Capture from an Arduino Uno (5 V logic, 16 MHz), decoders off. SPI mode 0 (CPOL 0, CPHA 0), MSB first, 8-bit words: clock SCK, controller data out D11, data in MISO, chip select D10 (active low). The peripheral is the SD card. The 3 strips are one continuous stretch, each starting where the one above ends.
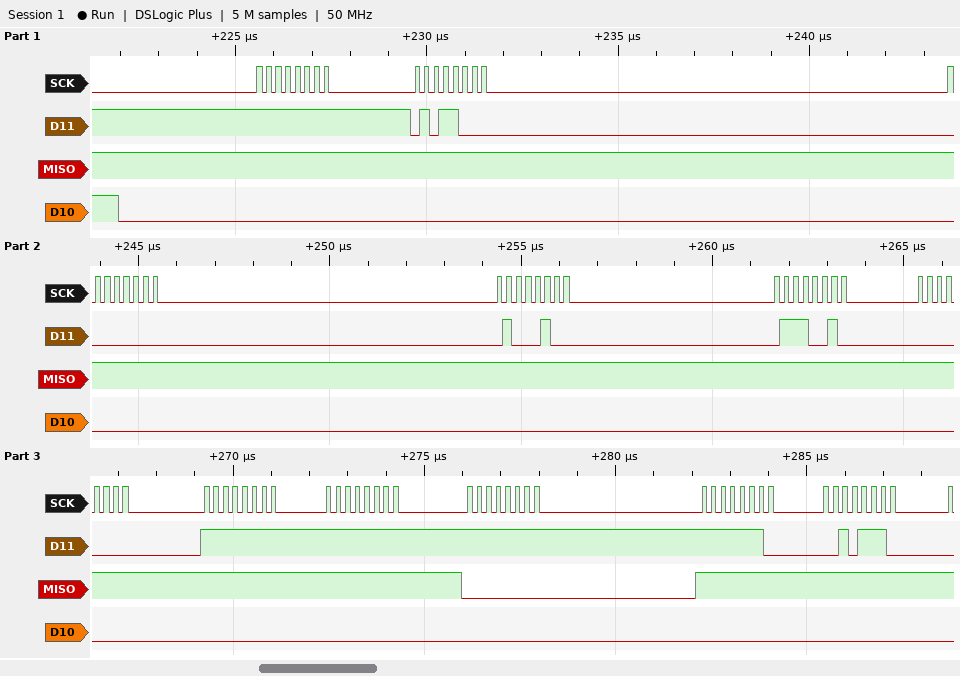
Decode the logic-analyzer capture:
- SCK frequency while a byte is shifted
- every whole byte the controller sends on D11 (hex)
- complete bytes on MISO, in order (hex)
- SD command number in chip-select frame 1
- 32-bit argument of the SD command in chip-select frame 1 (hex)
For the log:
4 MHz
FF 58 00 44 72 00 FF FF FF FE 2E
FF FF FF FF FF FF FF FF 00 FF FF
CMD24
0x00447200
